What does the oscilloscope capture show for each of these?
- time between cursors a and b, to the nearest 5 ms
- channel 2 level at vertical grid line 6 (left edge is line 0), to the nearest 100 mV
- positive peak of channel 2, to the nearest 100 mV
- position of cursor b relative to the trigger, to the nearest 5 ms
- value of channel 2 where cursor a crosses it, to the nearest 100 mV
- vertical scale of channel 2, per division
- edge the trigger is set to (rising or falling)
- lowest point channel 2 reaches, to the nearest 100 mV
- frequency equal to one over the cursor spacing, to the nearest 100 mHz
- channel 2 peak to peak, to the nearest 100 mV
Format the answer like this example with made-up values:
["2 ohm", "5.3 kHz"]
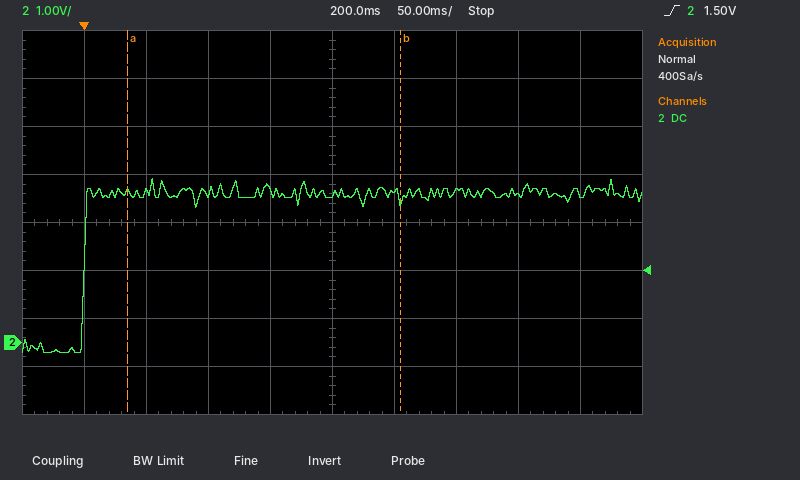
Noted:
["220 ms", "3.2 V", "3.4 V", "+255 ms", "3.1 V", "1 V", "rising", "-200 mV", "4.5 Hz", "3.6 V"]
